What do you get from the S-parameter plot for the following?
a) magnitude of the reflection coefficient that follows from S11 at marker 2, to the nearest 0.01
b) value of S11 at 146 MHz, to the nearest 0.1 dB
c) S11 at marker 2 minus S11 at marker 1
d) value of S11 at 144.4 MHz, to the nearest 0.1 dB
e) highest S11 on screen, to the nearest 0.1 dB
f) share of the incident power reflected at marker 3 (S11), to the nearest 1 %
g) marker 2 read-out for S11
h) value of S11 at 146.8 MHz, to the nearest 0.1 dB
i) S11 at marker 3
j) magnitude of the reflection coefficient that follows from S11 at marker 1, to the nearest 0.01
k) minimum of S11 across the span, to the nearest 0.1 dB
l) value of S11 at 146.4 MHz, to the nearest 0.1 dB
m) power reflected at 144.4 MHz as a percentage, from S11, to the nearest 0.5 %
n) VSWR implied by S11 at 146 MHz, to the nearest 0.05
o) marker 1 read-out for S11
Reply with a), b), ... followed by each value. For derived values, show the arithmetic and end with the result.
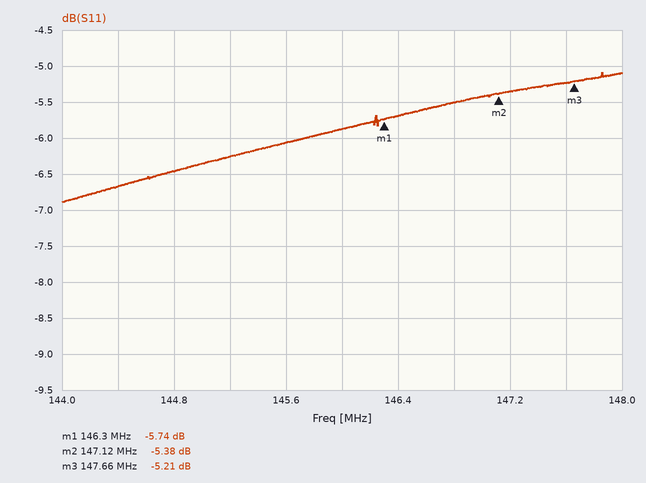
a) 10^(-5.38/20) ≈ 0.54
b) -5.9 dB
c) -5.38 − (-5.74) = 0.36 dB
d) -6.7 dB
e) -5.1 dB
f) 10^(-5.21/10) ≈ 30 %
g) -5.38 dB
h) -5.5 dB
i) -5.21 dB
j) 10^(-5.74/20) ≈ 0.52
k) -6.9 dB
l) -5.7 dB
m) 10^(-6.7/10) ≈ 21.4 %, so 21.5 % to the nearest 0.5 %
n) |Γ| = 10^(-5.9/20) = 0.5070; VSWR = (1 + 0.5070)/(1 − 0.5070) ≈ 3.06, so 3.05 to the nearest 0.05
o) -5.74 dB
